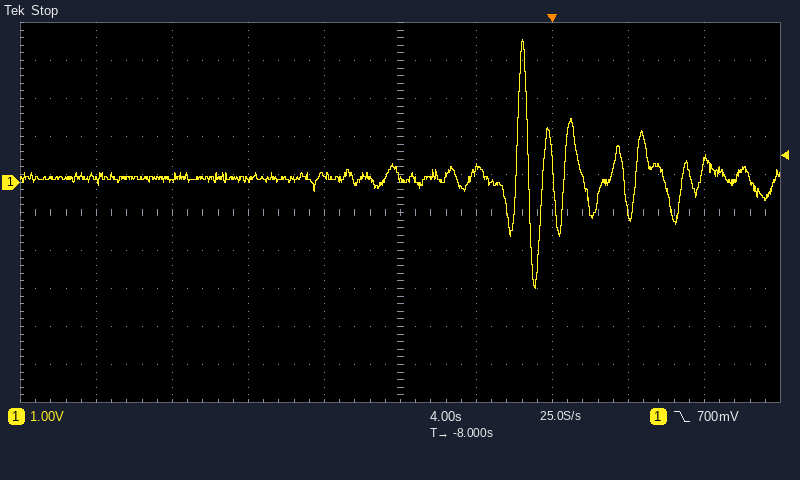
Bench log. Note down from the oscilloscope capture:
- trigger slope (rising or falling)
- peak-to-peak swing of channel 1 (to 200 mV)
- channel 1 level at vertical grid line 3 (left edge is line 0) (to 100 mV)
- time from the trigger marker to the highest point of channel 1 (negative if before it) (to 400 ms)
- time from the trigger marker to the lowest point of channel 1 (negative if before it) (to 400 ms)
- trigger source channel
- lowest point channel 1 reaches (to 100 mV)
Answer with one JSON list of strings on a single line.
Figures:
["falling", "6.6 V", "100 mV", "-1.6 s", "-800 ms", "channel 1", "-2.8 V"]
